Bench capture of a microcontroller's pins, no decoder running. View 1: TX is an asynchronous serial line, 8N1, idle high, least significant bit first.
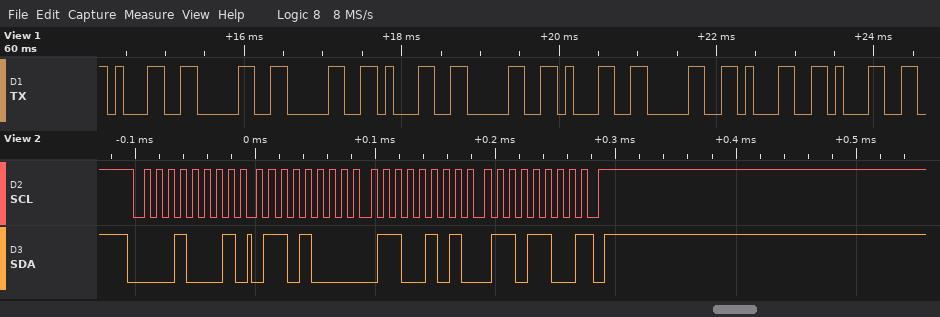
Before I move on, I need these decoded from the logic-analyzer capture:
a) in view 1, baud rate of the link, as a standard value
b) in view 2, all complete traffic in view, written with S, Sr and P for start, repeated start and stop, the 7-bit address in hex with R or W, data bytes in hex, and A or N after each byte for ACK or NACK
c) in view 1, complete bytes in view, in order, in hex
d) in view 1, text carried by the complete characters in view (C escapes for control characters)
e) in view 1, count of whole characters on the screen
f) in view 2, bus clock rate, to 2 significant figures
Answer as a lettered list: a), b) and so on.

a) 9600 baud
b) S 08R A 68 A 65 A 6C N P
c) 0x31 0x30 0x30 0x31 0x30 0x31 0x30 0x31 0x31
d) "100101011"
e) 9
f) 100 kHz
